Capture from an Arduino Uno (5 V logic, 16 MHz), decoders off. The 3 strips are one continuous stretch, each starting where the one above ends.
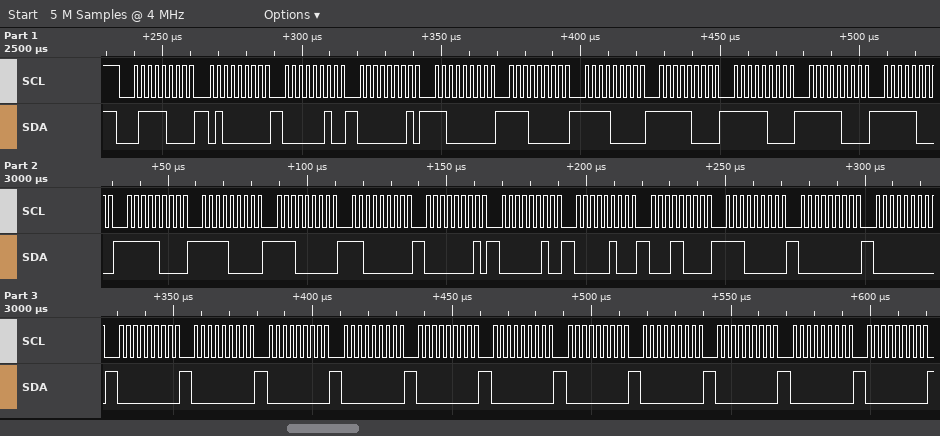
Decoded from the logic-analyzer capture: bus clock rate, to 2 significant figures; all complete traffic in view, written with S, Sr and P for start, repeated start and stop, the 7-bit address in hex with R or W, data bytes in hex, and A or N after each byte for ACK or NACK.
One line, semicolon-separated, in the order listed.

400 kHz; S 3CW A 40 A 02 A 01 A C0 A E0 A F0 A F8 A F8 A F8 A F8 A F8 A F0 A E0 A C0 A 01 A 02 A 04 A 18 A E0 A 00 A 00 A 00 A 00 A 00 A 00 A 00 A 00 A 00 A 00 A 00 A 00 A 00 A
